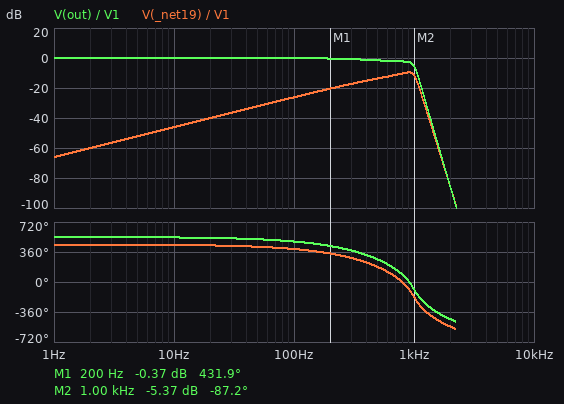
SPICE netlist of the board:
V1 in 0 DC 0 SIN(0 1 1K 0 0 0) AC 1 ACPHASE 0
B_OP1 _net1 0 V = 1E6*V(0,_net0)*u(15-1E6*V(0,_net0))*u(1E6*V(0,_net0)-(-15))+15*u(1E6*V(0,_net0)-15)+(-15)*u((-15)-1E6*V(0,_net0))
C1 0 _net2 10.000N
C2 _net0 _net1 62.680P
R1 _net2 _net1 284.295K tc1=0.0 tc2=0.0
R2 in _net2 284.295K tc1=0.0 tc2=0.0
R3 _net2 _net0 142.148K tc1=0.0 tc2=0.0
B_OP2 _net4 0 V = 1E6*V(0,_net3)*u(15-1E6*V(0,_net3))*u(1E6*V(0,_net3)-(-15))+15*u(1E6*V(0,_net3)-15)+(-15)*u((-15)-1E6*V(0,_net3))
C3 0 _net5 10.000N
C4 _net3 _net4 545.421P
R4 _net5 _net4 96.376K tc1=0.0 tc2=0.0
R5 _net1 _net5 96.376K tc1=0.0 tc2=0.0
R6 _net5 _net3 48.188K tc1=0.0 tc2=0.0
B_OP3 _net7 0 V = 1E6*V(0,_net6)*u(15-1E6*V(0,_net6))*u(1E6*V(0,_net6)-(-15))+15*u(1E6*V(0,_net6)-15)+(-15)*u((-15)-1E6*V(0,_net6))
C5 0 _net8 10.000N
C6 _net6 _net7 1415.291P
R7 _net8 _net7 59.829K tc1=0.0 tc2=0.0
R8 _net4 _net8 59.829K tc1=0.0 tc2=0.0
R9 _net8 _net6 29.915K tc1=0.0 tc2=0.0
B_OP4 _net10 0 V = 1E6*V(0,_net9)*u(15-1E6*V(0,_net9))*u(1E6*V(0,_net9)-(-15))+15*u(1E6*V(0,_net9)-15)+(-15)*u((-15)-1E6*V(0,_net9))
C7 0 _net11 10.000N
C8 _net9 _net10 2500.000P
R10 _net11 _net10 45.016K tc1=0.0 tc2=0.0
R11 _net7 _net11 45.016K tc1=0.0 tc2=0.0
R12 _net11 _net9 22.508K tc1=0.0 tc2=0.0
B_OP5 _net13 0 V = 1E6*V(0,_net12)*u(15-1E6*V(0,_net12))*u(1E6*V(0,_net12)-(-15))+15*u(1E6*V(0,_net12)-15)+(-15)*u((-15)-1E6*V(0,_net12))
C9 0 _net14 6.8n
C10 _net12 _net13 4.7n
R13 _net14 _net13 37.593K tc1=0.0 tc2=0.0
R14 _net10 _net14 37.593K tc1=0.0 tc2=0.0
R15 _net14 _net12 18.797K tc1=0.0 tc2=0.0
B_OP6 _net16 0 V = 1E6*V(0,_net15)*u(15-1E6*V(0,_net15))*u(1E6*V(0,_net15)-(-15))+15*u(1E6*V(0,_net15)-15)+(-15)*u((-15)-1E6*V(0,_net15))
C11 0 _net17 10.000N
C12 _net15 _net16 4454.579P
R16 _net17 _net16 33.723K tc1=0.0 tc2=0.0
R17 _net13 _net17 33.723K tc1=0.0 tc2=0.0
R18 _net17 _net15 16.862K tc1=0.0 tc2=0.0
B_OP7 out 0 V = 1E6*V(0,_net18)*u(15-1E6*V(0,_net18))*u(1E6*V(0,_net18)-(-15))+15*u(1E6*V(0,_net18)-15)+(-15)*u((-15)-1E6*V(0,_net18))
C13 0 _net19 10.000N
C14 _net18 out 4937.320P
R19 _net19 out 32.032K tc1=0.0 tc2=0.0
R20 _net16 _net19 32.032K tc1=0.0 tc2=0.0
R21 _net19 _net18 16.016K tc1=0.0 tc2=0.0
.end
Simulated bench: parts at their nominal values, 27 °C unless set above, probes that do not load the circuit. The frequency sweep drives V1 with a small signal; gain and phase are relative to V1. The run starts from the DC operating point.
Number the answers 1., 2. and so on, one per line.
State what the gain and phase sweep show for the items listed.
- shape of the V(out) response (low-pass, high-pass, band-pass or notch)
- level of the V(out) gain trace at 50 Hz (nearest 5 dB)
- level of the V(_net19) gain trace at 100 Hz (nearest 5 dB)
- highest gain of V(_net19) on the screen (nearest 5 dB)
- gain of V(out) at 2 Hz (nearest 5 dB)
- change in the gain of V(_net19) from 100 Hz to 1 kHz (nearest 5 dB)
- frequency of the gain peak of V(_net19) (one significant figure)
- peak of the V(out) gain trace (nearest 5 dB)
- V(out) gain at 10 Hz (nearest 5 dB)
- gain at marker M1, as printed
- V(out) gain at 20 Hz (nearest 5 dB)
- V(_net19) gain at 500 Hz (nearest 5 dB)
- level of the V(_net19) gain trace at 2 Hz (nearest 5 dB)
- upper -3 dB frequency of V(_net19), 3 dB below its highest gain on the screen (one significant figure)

1. low-pass
2. 0 dB
3. -25 dB
4. -10 dB
5. 0 dB
6. 15 dB
7. 900 Hz
8. 0 dB
9. 0 dB
10. -0.37 dB
11. 0 dB
12. -15 dB
13. -60 dB
14. 1 kHz
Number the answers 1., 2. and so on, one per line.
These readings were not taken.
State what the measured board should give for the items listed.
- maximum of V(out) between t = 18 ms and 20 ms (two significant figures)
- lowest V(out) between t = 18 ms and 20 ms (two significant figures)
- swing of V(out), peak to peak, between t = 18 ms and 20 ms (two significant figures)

1. 540 mV
2. -540 mV
3. 1.1 V
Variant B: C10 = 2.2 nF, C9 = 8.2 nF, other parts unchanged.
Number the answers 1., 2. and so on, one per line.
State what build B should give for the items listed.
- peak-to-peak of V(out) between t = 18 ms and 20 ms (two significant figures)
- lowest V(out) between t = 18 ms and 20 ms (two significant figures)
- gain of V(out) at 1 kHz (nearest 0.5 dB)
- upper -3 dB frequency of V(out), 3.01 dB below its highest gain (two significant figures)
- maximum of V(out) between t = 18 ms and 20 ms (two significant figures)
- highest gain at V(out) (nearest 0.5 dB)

1. 2.1 V
2. -1.0 V
3. 0.5 dB
4. 1.0 kHz
5. 1.0 V
6. 2.5 dB
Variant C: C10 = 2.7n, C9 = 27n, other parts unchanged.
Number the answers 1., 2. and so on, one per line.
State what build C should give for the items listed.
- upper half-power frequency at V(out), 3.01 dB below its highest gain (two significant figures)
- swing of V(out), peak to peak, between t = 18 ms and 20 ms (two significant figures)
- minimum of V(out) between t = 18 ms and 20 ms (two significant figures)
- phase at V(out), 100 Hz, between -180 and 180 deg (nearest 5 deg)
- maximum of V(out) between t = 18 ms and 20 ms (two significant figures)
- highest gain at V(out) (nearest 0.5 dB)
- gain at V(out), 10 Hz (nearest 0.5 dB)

1. 930 Hz
2. 1.5 V
3. -730 mV
4. 130 deg
5. 730 mV
6. 3.5 dB
7. 0 dB
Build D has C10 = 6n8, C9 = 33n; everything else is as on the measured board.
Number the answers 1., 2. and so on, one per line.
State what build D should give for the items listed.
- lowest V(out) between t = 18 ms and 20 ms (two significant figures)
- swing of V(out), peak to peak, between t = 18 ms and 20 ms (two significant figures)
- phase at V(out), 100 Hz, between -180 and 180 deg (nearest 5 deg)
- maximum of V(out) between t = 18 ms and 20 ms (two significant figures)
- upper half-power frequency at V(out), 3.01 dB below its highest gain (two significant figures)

1. -190 mV
2. 390 mV
3. 120 deg
4. 190 mV
5. 460 Hz
